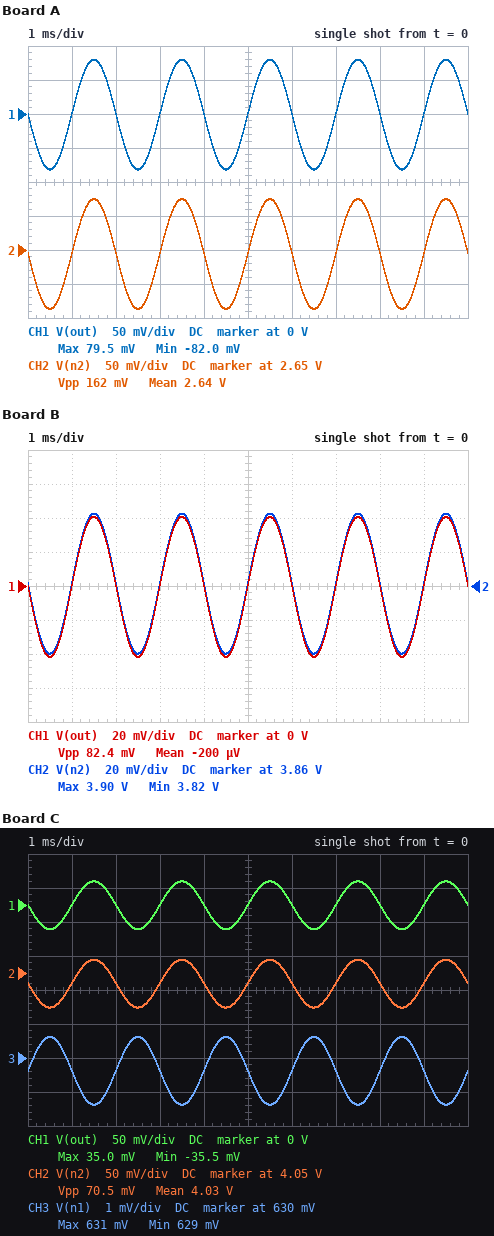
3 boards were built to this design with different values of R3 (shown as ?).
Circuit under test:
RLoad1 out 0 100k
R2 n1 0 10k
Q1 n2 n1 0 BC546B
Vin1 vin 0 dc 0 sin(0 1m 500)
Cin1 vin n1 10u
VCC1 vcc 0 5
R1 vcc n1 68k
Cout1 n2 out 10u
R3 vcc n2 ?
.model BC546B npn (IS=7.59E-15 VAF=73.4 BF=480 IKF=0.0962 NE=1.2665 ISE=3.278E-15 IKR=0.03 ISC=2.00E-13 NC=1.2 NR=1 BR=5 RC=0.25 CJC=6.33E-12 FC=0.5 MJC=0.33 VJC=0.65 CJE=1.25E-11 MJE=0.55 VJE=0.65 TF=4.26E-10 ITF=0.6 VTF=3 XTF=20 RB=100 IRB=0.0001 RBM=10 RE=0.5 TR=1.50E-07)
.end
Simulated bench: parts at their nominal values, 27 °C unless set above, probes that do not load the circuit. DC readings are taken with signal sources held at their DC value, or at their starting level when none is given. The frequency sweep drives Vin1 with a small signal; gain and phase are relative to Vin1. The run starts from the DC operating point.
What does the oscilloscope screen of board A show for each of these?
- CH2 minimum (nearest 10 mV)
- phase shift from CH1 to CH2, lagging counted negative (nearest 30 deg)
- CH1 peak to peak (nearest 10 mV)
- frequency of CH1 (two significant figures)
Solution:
2.56 V
0 deg
160 mV
500 Hz
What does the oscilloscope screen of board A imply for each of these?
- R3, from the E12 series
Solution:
8.2 kΩ
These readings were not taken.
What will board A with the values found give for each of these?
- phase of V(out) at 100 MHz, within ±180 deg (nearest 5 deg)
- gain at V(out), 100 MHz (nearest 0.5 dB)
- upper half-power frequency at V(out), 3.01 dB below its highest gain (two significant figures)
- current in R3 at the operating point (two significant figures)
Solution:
35 deg
4.0 dB
2.5 MHz
290 µA
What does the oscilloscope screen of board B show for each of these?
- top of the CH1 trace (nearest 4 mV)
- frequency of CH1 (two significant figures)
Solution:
40 mV
500 Hz
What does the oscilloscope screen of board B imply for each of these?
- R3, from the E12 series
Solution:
3.9 kΩ
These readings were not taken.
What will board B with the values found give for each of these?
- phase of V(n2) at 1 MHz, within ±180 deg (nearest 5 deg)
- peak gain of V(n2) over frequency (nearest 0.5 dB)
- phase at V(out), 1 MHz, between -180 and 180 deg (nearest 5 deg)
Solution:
170 deg
32.5 dB
170 deg
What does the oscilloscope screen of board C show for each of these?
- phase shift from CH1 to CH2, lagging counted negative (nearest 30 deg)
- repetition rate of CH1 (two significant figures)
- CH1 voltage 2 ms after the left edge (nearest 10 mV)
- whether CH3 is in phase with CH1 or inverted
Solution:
0 deg
500 Hz
0 V
inverted
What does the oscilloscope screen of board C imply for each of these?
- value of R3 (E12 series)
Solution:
3.3 kΩ
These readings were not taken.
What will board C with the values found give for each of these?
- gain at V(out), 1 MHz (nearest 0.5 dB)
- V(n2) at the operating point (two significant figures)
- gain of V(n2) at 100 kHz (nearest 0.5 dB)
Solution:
31.0 dB
4.0 V
31.0 dB
